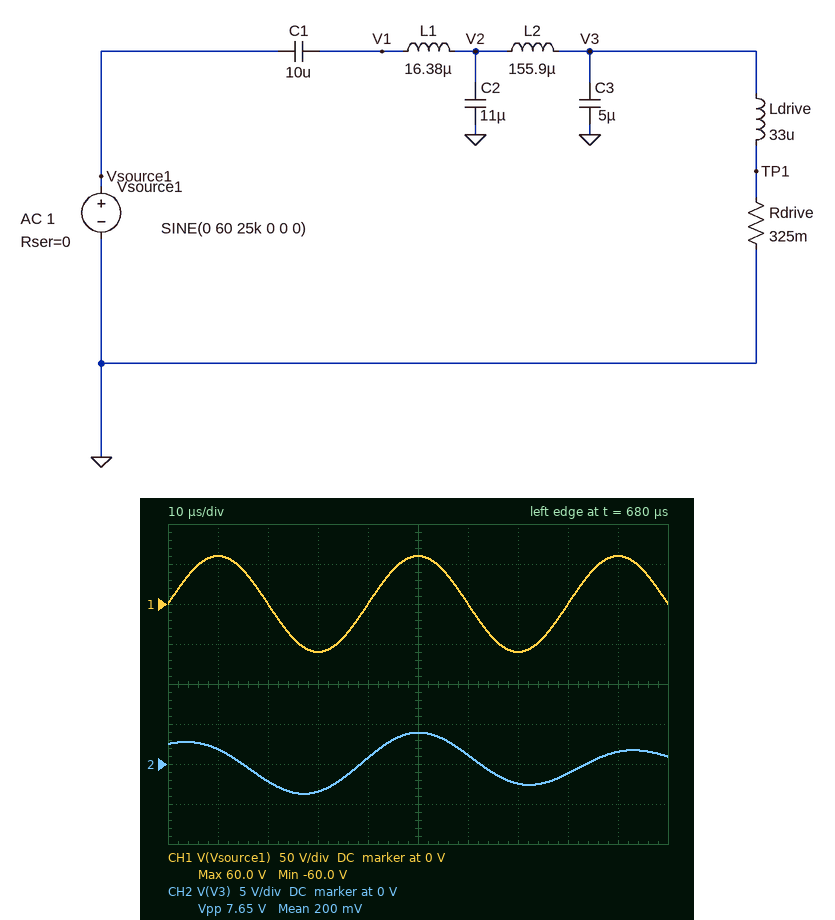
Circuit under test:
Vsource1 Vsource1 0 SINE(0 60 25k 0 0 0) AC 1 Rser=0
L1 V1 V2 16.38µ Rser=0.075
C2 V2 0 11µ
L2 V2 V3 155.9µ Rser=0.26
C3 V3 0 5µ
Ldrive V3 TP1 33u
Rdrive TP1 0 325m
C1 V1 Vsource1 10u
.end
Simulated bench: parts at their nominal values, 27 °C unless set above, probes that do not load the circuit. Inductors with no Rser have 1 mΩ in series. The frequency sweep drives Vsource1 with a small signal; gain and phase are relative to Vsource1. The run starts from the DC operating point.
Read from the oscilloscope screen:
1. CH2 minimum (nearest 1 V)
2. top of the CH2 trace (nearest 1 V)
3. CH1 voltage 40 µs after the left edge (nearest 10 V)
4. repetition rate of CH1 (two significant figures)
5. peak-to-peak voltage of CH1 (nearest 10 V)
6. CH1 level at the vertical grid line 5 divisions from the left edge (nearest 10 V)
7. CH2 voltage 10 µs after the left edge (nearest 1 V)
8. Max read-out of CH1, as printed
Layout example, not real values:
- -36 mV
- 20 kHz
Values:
- -4 V
- 4 V
- 0 V
- 25 kHz
- 120 V
- 60 V
- 2 V
- 60.0 V
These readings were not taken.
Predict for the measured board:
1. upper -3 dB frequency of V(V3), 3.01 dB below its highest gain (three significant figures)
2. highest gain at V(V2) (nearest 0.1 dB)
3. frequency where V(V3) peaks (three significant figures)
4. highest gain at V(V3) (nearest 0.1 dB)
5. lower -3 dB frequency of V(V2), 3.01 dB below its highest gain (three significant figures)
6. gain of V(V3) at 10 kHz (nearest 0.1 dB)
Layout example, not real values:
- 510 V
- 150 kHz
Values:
- 17.7 kHz
- 21.1 dB
- 17.4 kHz
- 9.8 dB
- 17.1 kHz
- -11.1 dB
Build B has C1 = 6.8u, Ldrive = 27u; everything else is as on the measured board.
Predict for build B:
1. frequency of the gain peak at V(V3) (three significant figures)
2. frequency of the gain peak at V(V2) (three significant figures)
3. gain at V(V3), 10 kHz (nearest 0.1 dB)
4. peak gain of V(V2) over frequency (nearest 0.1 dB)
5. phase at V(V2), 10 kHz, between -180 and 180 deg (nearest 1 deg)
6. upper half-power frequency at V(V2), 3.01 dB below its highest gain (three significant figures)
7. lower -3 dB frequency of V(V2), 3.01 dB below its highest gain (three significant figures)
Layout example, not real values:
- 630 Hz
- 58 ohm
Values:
- 19.3 kHz
- 19.4 kHz
- -16.4 dB
- 20.2 dB
- -1 deg
- 19.7 kHz
- 19.0 kHz
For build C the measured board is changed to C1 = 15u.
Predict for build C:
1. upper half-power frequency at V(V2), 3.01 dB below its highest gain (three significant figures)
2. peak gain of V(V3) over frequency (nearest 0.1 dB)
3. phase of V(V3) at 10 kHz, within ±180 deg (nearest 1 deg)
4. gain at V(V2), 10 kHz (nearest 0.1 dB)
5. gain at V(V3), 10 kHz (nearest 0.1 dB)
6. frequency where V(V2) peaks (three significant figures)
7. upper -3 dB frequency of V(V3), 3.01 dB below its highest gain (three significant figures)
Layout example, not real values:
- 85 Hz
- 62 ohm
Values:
- 16.4 kHz
- 14.5 dB
- -18 deg
- -0.2 dB
- -8.6 dB
- 16.0 kHz
- 16.3 kHz
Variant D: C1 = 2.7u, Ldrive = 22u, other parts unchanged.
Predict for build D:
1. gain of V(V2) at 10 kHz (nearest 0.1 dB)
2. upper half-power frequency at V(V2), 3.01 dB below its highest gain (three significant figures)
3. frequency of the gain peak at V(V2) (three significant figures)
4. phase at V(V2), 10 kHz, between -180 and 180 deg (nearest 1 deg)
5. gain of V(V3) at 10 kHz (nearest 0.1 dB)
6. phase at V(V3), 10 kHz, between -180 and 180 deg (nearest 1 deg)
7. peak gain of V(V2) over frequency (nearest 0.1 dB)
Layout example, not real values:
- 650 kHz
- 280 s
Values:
- -12.0 dB
- 27.1 kHz
- 26.8 kHz
- 0 deg
- -25.8 dB
- -18 deg
- 17.3 dB
